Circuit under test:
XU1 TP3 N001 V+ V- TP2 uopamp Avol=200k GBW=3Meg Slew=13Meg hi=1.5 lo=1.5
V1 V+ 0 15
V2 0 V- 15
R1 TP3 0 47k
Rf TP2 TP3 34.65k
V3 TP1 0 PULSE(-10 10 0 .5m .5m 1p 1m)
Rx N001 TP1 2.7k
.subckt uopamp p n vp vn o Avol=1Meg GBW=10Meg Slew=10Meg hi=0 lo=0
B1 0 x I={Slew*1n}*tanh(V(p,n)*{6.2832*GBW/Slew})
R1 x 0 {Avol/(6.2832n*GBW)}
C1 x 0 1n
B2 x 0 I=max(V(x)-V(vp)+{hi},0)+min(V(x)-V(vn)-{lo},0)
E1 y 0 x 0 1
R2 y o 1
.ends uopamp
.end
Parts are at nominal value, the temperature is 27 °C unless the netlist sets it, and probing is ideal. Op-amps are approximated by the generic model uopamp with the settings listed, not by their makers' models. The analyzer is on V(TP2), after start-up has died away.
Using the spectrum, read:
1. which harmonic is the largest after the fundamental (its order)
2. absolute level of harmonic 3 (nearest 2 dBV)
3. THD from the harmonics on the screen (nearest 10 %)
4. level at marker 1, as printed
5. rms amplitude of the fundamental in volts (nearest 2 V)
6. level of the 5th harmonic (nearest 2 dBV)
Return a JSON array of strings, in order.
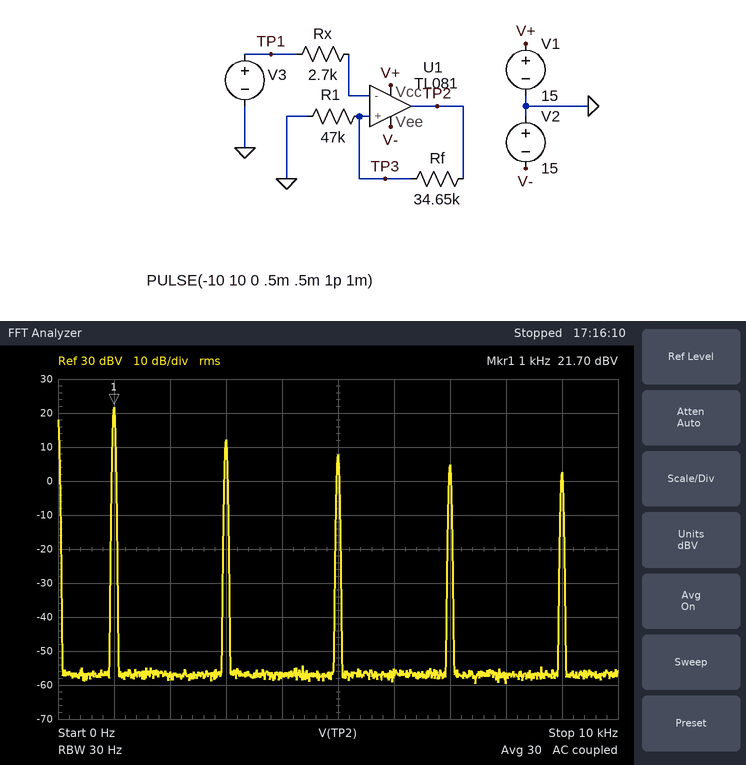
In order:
["3", "12 dBV", "40 %", "21.70 dBV", "12 V", "8 dBV"]
